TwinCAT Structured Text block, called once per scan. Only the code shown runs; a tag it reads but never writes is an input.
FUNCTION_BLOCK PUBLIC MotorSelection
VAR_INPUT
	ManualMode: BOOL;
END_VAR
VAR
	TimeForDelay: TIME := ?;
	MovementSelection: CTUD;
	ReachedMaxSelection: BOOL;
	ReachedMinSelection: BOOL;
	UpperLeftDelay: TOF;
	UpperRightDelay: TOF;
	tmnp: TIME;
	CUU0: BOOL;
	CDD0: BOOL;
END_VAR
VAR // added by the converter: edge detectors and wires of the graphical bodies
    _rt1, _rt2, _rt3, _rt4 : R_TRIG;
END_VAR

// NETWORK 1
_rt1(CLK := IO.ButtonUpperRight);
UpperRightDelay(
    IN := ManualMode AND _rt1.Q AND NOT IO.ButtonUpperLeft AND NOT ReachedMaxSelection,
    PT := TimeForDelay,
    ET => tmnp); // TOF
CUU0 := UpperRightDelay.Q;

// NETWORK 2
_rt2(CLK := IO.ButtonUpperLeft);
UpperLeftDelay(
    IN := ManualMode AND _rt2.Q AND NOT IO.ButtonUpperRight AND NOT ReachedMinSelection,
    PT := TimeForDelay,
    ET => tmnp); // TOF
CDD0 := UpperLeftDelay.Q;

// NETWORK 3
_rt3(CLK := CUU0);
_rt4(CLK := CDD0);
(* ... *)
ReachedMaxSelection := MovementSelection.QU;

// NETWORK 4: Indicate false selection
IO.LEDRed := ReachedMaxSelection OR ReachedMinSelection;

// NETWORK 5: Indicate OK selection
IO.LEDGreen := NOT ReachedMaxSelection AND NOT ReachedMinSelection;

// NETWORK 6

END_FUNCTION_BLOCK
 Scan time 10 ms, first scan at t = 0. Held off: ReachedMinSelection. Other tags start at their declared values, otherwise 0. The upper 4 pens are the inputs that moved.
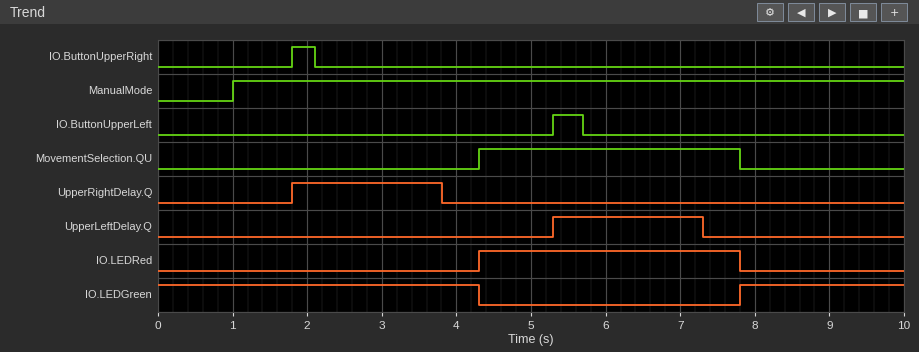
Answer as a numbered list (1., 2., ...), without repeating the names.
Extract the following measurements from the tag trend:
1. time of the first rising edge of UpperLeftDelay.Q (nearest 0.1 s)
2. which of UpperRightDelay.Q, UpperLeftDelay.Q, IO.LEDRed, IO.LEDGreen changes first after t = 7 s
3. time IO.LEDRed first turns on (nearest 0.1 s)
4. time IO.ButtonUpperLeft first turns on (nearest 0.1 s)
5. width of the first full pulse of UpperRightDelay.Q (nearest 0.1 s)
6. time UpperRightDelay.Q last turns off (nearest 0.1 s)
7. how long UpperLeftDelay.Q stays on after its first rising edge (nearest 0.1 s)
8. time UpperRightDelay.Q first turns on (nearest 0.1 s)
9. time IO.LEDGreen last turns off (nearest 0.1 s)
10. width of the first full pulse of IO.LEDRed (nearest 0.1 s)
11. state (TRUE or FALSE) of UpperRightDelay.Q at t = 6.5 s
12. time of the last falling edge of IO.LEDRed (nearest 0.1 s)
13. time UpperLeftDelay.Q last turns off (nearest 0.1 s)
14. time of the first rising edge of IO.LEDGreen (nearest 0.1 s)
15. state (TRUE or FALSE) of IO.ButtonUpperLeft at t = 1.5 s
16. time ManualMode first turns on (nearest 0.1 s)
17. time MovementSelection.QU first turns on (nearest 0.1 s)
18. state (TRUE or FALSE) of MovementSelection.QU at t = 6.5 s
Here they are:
1. 5.3 s
2. UpperLeftDelay.Q
3. 4.3 s
4. 5.3 s
5. 2.0 s
6. 3.8 s
7. 2.0 s
8. 1.8 s
9. 4.3 s
10. 3.5 s
11. FALSE
12. 7.8 s
13. 7.3 s
14. 7.8 s
15. FALSE
16. 1.0 s
17. 4.3 s
18. TRUE
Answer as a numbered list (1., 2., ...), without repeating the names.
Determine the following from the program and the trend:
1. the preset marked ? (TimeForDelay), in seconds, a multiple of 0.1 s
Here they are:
1. 2.0 s
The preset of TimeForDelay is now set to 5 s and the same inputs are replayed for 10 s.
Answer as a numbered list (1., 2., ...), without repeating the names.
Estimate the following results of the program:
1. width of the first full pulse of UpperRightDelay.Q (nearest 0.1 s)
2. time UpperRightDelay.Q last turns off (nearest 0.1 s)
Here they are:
1. 5.0 s
2. 6.8 s
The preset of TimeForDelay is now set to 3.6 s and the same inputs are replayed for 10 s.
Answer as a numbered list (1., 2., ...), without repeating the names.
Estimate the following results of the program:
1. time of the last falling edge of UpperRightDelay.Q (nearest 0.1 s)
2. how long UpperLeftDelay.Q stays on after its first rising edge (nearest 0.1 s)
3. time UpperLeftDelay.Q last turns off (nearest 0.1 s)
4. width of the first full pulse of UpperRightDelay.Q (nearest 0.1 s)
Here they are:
1. 5.4 s
2. 3.6 s
3. 8.9 s
4. 3.6 s
